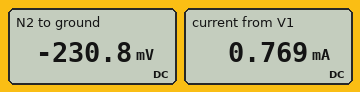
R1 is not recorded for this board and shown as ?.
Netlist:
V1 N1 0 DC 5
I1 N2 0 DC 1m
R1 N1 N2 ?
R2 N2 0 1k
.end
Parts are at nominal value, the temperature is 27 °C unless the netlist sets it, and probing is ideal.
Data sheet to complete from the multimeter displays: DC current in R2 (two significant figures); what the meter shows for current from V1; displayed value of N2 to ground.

230 µA
0.769 mA
-230.8 mV
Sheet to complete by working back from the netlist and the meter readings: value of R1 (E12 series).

6.8 kΩ
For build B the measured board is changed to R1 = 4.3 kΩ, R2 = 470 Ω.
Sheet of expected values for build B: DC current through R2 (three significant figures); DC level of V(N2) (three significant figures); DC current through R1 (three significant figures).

147 µA
69.0 mV
1.15 mA
